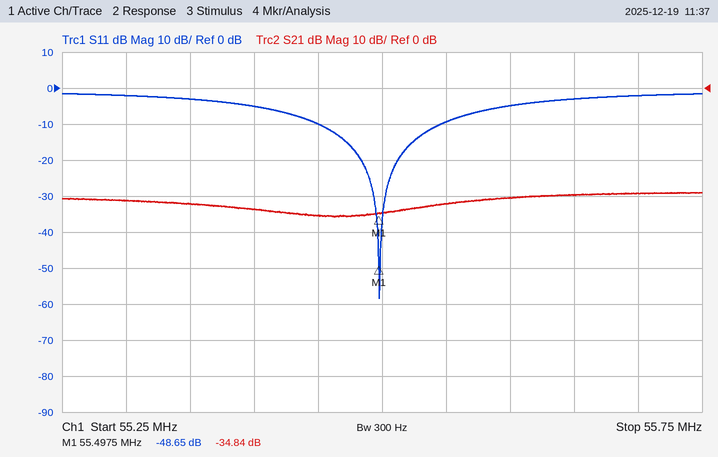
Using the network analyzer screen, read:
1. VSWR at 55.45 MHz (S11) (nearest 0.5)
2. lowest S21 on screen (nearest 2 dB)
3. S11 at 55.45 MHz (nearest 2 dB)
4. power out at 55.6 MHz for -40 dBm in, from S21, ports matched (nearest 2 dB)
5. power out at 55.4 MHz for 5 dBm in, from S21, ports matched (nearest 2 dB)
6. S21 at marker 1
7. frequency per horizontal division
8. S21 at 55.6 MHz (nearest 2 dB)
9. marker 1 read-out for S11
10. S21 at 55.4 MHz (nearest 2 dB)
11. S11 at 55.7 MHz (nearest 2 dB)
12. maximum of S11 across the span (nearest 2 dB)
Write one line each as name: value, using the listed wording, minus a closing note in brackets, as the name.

VSWR at 55.45 MHz (S11): 2.0
lowest S21 on screen: -36 dB
S11 at 55.45 MHz: -10 dB
power out at 55.6 MHz for -40 dBm in, from S21, ports matched: -70 dBm
power out at 55.4 MHz for 5 dBm in, from S21, ports matched: -28 dBm
S21 at marker 1: -34.84 dB
frequency per horizontal division: 50 kHz
S21 at 55.6 MHz: -30 dB
marker 1 read-out for S11: -48.65 dB
S21 at 55.4 MHz: -34 dB
S11 at 55.7 MHz: -2 dB
maximum of S11 across the span: -2 dB
